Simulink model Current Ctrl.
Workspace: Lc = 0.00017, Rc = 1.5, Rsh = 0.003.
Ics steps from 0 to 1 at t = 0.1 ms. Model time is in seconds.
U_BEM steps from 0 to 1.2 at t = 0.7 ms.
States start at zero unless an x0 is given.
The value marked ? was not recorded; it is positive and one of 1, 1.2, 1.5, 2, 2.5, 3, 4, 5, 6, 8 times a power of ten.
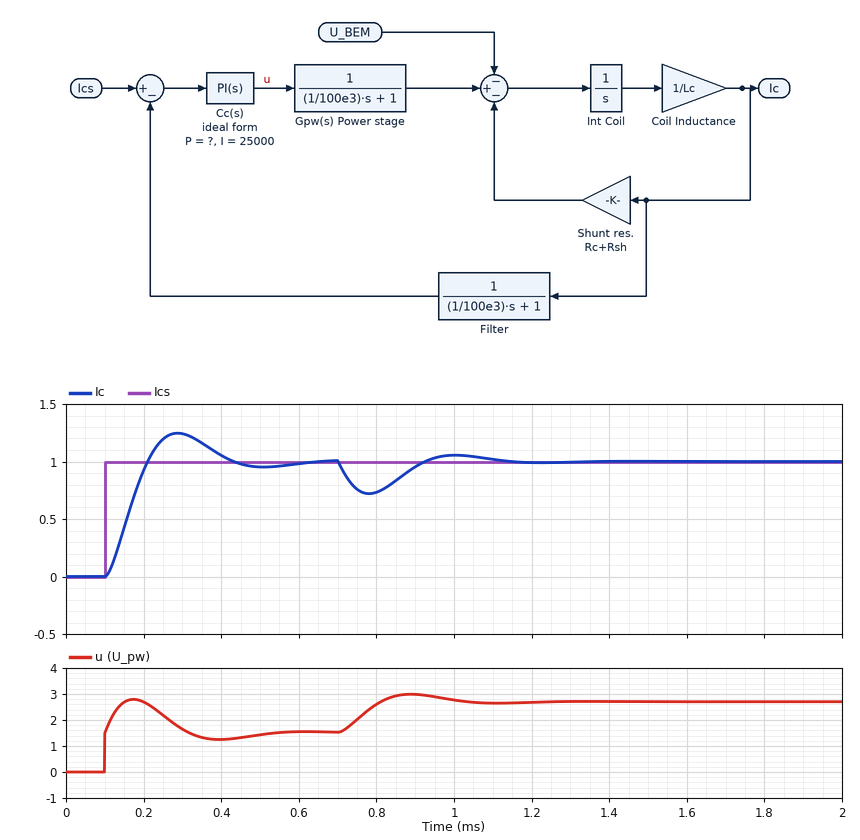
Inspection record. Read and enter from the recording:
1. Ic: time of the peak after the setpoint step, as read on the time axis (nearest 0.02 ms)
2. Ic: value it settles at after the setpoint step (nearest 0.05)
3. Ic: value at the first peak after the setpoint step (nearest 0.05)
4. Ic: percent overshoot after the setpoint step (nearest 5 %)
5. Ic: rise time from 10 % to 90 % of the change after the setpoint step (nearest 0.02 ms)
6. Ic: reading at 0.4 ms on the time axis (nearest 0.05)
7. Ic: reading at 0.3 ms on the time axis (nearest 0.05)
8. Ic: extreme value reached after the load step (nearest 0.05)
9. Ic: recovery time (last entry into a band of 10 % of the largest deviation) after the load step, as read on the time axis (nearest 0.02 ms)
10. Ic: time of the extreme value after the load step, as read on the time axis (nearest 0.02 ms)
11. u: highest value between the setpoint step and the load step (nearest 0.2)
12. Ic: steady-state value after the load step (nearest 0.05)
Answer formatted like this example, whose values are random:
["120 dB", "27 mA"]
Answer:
["0.28 ms", "1.00", "1.25", "25 %", "0.08 ms", "1.05", "1.25", "0.70", "1.08 ms", "0.78 ms", "2.8", "1.00"]
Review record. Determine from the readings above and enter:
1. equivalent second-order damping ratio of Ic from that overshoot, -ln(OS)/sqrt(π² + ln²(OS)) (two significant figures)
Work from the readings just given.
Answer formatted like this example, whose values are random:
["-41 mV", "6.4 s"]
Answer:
["0.40"]
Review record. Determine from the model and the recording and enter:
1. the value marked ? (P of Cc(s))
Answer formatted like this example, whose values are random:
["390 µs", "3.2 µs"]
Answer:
["1.5"]
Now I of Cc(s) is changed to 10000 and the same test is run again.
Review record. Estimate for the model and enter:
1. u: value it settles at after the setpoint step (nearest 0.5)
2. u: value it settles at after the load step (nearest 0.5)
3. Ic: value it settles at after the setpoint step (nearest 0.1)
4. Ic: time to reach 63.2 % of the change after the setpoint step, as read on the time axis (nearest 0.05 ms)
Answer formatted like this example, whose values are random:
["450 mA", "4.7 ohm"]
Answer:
["1.5", "2.5", "1.0", "0.20 ms"]
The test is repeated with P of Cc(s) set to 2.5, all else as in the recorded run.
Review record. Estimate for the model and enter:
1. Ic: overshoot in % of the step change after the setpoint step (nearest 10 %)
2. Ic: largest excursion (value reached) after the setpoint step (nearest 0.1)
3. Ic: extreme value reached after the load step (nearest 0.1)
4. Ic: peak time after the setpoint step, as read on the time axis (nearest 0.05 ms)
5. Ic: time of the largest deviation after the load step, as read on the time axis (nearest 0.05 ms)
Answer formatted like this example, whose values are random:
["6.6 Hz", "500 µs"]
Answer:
["30 %", "1.3", "0.8", "0.25 ms", "0.75 ms"]
